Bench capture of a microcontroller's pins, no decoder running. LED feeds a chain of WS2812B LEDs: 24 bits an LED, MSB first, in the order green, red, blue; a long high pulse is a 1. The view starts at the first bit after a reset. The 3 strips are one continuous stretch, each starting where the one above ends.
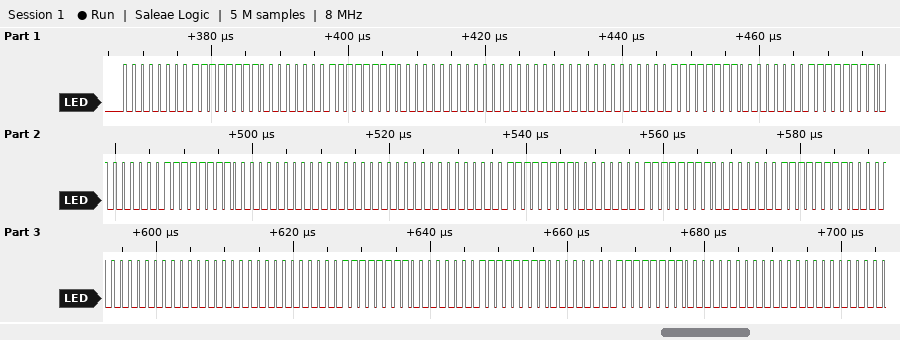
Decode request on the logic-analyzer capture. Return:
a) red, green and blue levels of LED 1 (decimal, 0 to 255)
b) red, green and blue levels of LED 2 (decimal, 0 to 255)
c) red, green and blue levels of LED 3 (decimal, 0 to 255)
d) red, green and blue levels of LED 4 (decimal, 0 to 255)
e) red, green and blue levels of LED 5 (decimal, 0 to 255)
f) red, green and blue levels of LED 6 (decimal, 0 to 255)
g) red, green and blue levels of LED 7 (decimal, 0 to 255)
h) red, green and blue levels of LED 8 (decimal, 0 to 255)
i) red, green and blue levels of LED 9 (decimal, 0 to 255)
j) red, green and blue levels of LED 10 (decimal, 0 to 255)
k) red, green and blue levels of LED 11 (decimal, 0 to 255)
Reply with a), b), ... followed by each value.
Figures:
a) 255, 0, 0
b) 0, 255, 0
c) 0, 0, 255
d) 255, 0, 0
e) 0, 255, 0
f) 0, 0, 255
g) 255, 0, 0
h) 0, 255, 0
i) 0, 0, 255
j) 255, 0, 0
k) 0, 255, 0
